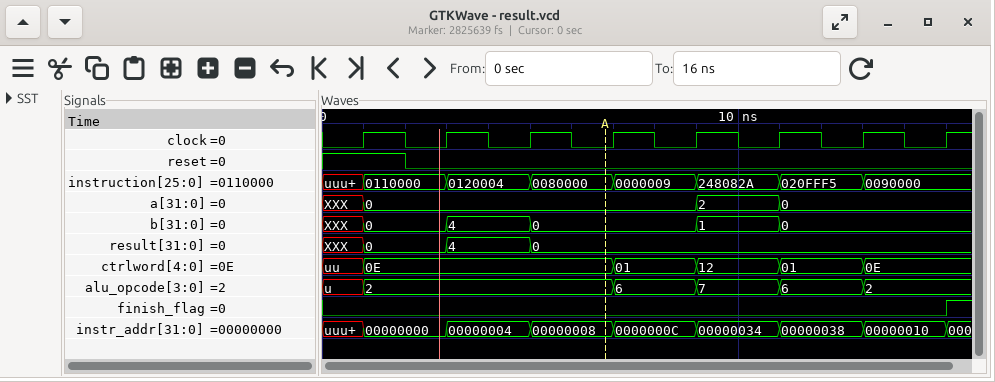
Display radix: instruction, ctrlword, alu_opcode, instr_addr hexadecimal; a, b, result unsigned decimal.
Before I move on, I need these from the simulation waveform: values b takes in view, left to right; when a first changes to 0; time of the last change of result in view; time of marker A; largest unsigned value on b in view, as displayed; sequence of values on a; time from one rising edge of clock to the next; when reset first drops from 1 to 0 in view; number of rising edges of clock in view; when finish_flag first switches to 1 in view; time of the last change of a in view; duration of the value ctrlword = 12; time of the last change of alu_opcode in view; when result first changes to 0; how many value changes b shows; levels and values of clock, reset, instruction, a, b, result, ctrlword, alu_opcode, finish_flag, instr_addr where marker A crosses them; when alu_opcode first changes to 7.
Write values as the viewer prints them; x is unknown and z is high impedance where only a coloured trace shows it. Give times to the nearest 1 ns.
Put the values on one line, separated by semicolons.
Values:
XXX, 0, 4, 0, 1, 0; 1 ns; 5 ns; 7 ns; 4; XXX, 0, 2, 0; 2 ns; 2 ns; 8; 15 ns; 11 ns; 2 ns; 13 ns; 1 ns; 5; clock=0, reset=0, instruction=0080000, a=0, b=0, result=0, ctrlword=0E, alu_opcode=2, finish_flag=0, instr_addr=00000008; 9 ns
